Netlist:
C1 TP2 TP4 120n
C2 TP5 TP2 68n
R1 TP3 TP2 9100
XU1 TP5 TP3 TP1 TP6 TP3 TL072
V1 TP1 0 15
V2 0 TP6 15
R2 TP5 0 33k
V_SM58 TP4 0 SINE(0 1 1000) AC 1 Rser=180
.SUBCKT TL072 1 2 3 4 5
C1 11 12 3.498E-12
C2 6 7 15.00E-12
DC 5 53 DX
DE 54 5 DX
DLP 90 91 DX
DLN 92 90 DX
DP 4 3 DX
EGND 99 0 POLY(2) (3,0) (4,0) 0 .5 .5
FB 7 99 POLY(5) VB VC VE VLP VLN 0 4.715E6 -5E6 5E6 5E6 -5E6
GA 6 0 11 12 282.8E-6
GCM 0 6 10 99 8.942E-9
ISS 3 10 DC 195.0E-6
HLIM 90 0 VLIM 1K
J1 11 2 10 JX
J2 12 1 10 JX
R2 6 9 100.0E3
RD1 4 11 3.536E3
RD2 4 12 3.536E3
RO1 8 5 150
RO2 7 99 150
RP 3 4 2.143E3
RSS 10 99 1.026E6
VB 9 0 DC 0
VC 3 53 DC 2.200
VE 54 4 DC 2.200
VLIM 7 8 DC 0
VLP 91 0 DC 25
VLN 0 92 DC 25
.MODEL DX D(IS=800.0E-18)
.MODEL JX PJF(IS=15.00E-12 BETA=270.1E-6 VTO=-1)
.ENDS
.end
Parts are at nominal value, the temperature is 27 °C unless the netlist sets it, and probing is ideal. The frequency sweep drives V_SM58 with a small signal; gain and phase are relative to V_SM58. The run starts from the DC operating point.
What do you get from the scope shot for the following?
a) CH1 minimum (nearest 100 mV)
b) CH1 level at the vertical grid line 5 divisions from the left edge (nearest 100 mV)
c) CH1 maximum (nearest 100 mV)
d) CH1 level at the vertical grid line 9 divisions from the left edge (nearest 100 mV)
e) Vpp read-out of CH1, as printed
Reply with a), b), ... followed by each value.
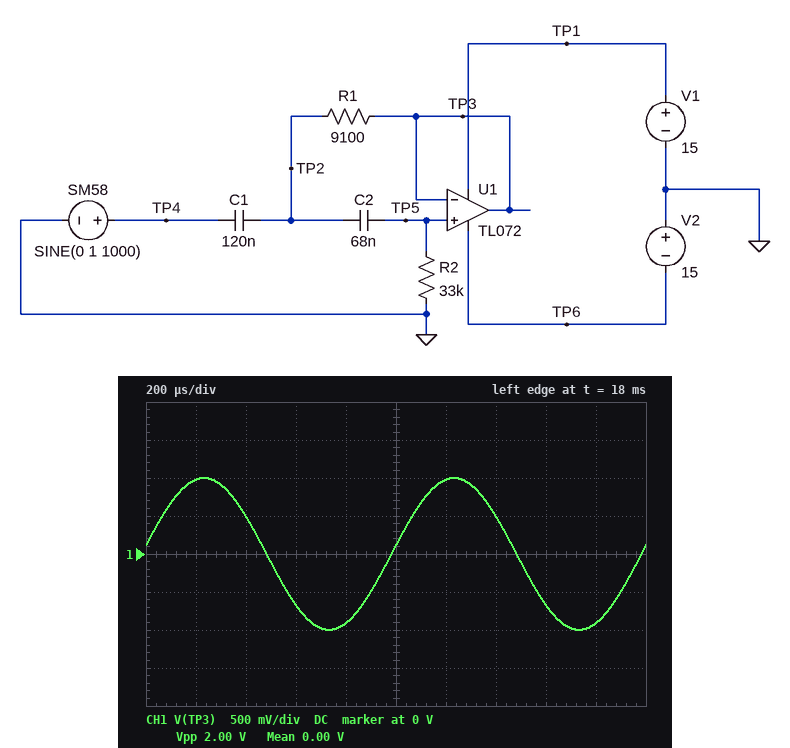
a) -1.0 V
b) 100 mV
c) 1.0 V
d) -900 mV
e) 2.00 V
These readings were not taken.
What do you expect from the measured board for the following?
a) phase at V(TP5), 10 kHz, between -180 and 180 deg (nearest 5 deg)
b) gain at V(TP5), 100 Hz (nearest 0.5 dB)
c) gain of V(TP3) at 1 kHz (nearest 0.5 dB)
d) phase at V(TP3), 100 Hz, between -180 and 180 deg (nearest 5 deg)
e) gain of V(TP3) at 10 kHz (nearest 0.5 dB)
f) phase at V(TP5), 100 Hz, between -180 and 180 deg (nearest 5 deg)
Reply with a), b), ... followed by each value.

a) 0 deg
b) -1.0 dB
c) 0 dB
d) 90 deg
e) 0 dB
f) 90 deg
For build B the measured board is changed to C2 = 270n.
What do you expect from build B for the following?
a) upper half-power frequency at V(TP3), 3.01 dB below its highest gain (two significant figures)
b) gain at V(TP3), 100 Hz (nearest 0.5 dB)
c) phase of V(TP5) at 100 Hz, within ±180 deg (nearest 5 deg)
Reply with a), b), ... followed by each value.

a) 4.3 MHz
b) 0.5 dB
c) 40 deg
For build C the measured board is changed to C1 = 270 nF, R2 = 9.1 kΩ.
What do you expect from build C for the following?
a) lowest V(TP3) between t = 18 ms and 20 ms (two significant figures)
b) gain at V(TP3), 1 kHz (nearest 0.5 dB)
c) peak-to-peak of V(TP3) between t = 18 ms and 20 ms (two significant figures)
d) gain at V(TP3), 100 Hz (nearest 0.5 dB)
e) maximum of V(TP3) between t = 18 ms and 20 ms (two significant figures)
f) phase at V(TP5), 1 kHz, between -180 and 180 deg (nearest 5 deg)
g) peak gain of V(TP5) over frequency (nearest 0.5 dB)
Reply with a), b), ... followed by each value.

a) -950 mV
b) -0.5 dB
c) 1.9 V
d) -10.5 dB
e) 950 mV
f) 20 deg
g) 0 dB
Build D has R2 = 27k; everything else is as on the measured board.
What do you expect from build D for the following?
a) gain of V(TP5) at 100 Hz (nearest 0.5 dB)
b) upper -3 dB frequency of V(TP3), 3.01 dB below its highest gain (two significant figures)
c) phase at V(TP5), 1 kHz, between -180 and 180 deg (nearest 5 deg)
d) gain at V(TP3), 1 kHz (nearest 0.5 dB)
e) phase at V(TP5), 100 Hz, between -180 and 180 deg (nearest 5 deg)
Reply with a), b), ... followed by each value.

a) -3.0 dB
b) 4.5 MHz
c) 10 deg
d) 0 dB
e) 100 deg
